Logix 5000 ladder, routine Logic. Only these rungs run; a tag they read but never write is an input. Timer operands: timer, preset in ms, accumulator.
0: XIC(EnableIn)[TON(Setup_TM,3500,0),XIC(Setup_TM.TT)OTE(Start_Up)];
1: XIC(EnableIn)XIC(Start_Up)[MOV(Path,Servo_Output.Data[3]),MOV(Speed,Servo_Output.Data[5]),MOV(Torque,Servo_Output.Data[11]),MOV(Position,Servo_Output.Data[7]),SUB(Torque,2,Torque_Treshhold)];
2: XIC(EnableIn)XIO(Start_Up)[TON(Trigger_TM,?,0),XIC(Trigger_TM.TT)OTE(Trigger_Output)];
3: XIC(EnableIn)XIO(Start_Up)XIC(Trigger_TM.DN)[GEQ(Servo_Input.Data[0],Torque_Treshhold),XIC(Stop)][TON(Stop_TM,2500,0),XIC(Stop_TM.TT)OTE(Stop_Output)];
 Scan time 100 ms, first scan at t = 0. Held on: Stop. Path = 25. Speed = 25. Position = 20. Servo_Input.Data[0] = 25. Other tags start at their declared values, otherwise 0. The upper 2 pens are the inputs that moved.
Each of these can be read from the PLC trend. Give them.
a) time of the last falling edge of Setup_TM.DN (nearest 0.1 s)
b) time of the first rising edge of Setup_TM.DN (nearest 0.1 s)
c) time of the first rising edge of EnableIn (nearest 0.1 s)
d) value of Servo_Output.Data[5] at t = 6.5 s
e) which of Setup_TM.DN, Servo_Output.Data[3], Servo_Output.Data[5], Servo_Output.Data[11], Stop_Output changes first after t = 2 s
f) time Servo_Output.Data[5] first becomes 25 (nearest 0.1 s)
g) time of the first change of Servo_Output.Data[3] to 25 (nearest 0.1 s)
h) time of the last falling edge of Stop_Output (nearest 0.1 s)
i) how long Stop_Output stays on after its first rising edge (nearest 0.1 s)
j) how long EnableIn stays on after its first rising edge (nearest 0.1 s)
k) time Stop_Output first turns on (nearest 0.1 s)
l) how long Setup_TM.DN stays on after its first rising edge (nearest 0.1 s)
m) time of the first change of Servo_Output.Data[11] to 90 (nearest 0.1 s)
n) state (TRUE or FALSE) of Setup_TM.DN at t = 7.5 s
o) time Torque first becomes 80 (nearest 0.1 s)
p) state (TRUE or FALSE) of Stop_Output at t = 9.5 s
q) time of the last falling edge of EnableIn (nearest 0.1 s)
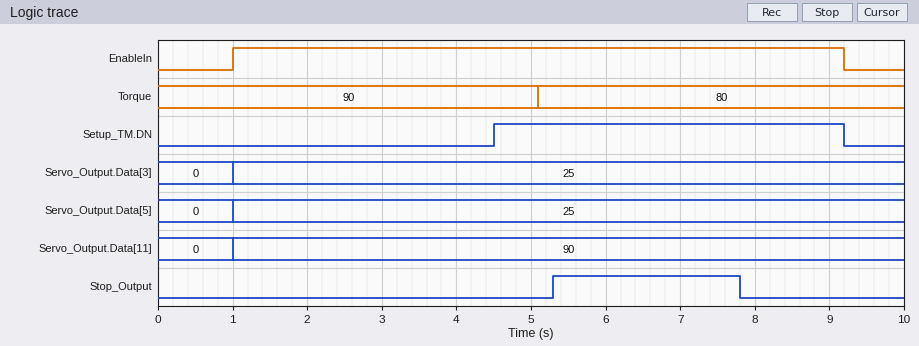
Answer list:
9.2 s
4.5 s
1.0 s
25
Setup_TM.DN
1.0 s
1.0 s
7.8 s
2.5 s
8.2 s
5.3 s
4.7 s
1.0 s
TRUE
5.1 s
FALSE
9.2 s
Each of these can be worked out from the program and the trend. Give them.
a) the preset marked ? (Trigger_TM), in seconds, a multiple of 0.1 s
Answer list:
0.8 s
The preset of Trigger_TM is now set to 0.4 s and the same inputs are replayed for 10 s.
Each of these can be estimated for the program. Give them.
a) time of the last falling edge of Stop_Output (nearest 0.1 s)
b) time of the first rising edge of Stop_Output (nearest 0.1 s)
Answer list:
7.4 s
4.9 s
